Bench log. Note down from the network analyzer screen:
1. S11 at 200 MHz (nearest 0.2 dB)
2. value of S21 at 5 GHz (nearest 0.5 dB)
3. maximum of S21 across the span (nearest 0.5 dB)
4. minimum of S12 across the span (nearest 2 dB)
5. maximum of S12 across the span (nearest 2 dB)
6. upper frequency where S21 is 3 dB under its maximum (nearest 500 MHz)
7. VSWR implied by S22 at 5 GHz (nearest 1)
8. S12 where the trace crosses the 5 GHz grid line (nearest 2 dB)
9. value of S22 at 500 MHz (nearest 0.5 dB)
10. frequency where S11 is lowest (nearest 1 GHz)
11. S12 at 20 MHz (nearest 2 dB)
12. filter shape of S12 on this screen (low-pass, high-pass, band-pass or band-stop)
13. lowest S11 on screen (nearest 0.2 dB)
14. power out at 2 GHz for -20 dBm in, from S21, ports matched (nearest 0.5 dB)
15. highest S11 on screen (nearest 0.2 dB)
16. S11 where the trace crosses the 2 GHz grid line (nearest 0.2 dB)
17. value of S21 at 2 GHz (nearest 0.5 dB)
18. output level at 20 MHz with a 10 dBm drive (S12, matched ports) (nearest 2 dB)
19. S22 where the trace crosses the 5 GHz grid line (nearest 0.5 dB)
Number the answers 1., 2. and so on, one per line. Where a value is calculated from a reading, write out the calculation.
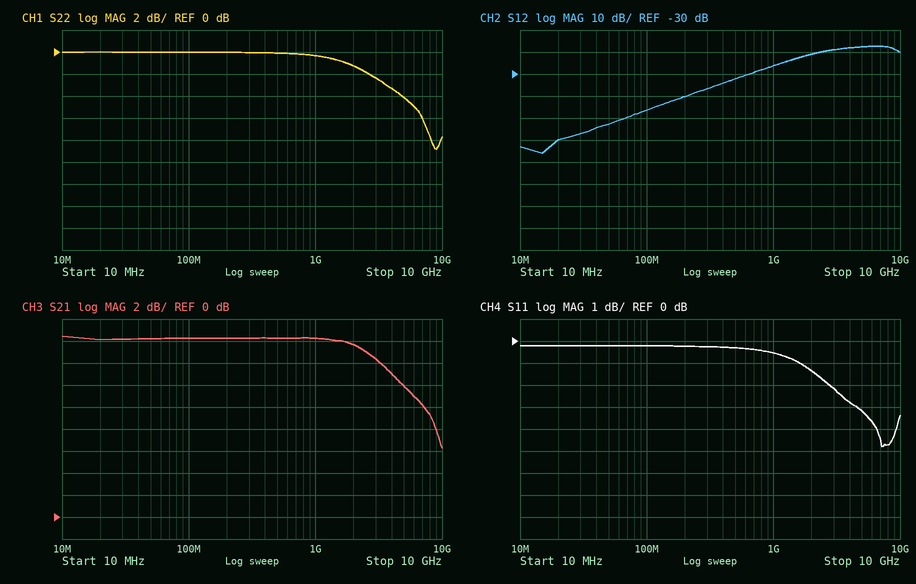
1. -0.2 dB
2. 12.0 dB
3. 16.5 dB
4. -66 dB
5. -18 dB
6. 3.5 GHz
7. |Γ| = 10^(-4/20) = 0.6310; VSWR = (1 + 0.6310)/(1 − 0.6310) ≈ 4
8. -18 dB
9. 0.0 dB
10. 7 GHz
11. -60 dB
12. high-pass
13. -4.8 dB
14. -20 dBm + (15.5 dB) = -4.5 dBm
15. -0.2 dB
16. -1.4 dB
17. 15.5 dB
18. 10 dBm + (-60 dB) = -50 dBm
19. -4.0 dB
